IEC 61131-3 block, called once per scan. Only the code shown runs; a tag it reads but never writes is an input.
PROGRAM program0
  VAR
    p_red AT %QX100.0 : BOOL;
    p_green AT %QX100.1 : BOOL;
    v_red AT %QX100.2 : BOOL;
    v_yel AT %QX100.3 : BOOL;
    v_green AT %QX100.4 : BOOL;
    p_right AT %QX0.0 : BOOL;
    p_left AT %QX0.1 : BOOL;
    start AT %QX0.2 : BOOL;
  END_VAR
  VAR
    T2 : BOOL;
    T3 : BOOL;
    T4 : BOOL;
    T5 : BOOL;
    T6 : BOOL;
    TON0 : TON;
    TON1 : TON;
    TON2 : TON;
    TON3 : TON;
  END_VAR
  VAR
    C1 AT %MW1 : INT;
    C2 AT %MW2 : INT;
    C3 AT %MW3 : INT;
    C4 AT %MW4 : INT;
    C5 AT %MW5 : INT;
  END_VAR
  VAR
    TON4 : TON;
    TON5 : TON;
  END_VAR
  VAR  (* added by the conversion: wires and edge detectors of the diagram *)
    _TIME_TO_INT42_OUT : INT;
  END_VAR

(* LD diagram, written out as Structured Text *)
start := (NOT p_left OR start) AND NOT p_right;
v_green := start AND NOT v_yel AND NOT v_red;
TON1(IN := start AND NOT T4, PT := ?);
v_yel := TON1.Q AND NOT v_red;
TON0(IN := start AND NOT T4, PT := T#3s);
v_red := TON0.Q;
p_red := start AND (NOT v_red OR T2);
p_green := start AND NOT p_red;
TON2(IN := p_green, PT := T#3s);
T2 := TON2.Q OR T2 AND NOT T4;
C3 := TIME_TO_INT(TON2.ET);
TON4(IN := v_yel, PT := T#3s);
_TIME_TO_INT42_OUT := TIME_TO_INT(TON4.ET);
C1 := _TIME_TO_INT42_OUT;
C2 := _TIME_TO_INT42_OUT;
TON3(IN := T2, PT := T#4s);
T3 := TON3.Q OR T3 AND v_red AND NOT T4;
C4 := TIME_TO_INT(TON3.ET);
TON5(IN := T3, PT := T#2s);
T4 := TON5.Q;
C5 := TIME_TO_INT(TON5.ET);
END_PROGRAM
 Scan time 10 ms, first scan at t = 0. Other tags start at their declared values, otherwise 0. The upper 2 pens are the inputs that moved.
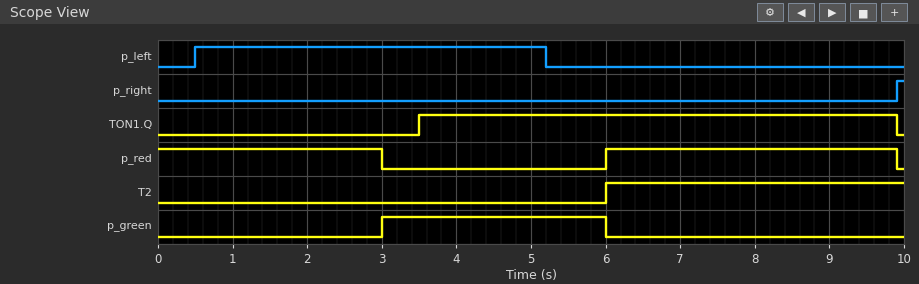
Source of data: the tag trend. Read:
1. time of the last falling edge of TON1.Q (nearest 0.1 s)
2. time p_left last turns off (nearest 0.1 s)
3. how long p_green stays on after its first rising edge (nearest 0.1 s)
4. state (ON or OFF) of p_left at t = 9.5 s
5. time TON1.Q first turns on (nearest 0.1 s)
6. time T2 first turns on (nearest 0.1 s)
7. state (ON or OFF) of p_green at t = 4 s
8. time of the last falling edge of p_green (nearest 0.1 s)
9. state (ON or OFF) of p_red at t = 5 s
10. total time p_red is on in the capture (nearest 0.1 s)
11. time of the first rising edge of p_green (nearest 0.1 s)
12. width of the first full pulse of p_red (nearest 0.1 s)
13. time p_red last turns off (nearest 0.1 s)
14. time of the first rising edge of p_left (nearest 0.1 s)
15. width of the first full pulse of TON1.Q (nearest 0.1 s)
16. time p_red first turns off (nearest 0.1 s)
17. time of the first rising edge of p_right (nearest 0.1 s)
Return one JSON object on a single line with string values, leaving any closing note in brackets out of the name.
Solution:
{"time of the last falling edge of TON1.Q": "9.9 s", "time p_left last turns off": "5.2 s", "how long p_green stays on after its first rising edge": "3.0 s", "state (ON or OFF) of p_left at t = 9.5 s": "OFF", "time TON1.Q first turns on": "3.5 s", "time T2 first turns on": "6.0 s", "state (ON or OFF) of p_green at t = 4 s": "ON", "time of the last falling edge of p_green": "6.0 s", "state (ON or OFF) of p_red at t = 5 s": "OFF", "total time p_red is on in the capture": "6.9 s", "time of the first rising edge of p_green": "3.0 s", "width of the first full pulse of p_red": "3.9 s", "time p_red last turns off": "9.9 s", "time of the first rising edge of p_left": "0.5 s", "width of the first full pulse of TON1.Q": "6.4 s", "time p_red first turns off": "3.0 s", "time of the first rising edge of p_right": "9.9 s"}
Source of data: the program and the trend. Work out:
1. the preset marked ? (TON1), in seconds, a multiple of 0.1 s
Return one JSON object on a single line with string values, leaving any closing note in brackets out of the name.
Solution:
{"the preset marked ? (TON1), in seconds, a multiple of 0.1 s": "3.5 s"}
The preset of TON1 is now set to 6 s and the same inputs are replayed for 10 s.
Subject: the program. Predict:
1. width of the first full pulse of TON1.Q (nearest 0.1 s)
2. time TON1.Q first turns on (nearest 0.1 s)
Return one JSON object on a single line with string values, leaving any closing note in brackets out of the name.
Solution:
{"width of the first full pulse of TON1.Q": "3.9 s", "time TON1.Q first turns on": "6.0 s"}
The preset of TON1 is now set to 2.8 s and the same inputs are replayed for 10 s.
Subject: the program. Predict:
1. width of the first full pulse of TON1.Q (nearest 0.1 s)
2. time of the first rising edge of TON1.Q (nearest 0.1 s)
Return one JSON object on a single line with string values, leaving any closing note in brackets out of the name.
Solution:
{"width of the first full pulse of TON1.Q": "7.1 s", "time of the first rising edge of TON1.Q": "2.8 s"}
